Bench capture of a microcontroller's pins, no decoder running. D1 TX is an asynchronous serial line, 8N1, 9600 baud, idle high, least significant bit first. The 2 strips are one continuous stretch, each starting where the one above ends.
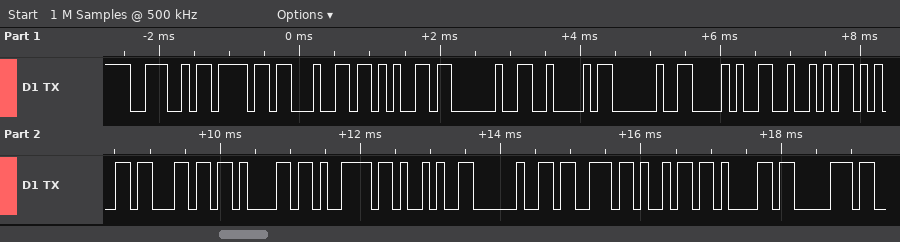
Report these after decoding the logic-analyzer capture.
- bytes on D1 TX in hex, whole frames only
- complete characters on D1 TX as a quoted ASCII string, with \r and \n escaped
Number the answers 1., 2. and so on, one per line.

1. 4E 6F 64 65 20 42 20 28 52 65 6C 61 79 29 20 73 69 61 70
2. "Node B (Relay) siap"
